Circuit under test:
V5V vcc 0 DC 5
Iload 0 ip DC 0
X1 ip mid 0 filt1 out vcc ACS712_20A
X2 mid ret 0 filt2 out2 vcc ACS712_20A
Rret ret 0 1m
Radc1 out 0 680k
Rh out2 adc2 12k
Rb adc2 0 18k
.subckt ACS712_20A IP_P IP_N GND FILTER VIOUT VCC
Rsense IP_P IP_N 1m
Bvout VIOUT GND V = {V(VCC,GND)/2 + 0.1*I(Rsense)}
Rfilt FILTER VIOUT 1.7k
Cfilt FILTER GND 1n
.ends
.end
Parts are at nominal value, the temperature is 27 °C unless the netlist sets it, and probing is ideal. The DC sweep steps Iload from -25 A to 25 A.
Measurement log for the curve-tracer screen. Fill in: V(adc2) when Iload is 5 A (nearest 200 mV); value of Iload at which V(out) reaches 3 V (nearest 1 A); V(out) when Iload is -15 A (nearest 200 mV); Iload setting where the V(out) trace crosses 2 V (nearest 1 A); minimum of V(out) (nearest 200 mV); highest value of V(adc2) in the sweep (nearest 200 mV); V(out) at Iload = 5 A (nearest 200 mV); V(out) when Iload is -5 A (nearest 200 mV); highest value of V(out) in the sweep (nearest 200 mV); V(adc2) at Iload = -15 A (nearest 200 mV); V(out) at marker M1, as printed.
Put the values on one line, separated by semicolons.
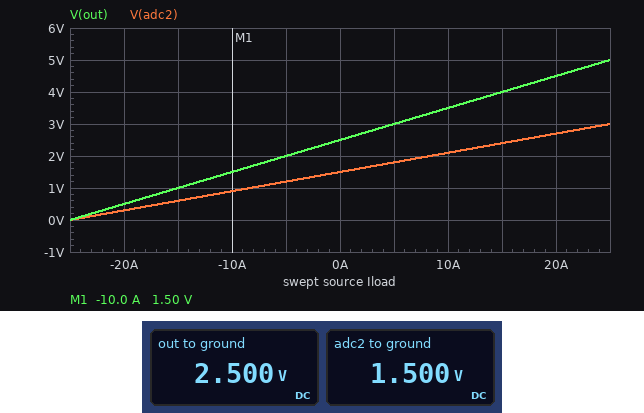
1.8 V; 5 A; 1.0 V; -5 A; 0 V; 3.0 V; 3.0 V; 2.0 V; 5.0 V; 600 mV; 1.50 V
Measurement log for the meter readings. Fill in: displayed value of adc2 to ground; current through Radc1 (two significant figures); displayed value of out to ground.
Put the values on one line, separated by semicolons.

1.500 V; 3.7 µA; 2.500 V
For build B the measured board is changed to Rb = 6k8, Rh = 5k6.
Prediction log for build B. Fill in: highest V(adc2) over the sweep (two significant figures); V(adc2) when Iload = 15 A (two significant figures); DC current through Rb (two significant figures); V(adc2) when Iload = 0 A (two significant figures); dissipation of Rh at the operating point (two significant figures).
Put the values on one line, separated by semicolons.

2.7 V; 2.2 V; 200 µA; 1.4 V; 230 µW
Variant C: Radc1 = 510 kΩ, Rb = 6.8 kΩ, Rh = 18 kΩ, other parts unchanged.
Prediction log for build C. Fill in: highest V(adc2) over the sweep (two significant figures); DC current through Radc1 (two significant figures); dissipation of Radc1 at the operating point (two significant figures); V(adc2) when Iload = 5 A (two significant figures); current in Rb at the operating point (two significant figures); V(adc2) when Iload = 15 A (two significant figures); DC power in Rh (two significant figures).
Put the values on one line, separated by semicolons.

1.4 V; 4.9 µA; 12 µW; 820 mV; 100 µA; 1.1 V; 180 µW
